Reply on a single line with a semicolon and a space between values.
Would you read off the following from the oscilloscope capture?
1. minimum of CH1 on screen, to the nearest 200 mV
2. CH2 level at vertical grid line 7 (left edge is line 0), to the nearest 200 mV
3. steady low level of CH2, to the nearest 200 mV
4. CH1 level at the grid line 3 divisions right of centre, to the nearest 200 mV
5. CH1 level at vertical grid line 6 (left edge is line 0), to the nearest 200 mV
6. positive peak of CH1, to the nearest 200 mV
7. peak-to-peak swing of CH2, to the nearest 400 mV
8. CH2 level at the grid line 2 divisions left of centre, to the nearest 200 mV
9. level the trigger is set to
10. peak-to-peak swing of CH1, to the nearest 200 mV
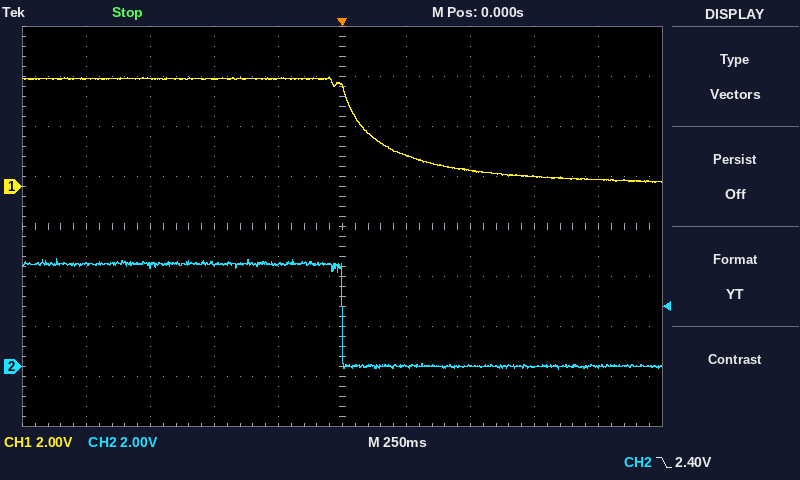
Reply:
200 mV; 0.0 V; 0.0 V; 400 mV; 1.2 V; 4.4 V; 4.4 V; 4.2 V; 2.40 V; 4.2 V
